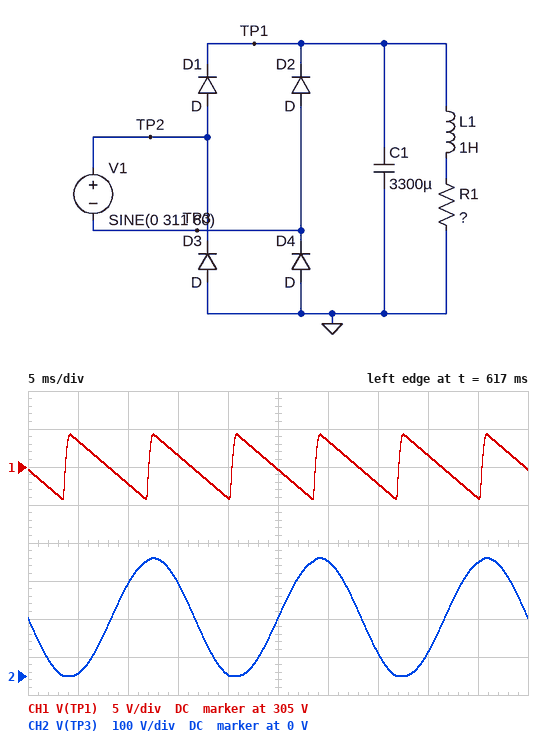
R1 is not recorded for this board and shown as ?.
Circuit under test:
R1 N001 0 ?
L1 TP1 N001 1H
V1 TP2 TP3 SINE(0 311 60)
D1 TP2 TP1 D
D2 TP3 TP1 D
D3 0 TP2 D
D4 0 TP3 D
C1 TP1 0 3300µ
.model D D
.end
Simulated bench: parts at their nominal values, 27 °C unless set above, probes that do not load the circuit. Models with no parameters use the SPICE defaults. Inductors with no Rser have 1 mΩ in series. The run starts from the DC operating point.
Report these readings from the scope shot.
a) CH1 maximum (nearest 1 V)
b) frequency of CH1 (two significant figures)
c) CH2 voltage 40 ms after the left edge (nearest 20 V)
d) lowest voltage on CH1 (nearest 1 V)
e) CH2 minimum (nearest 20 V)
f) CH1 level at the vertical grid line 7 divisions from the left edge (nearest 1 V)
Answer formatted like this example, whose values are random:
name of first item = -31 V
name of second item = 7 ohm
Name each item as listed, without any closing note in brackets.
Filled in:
CH1 maximum = 309 V
frequency of CH1 = 120 Hz
CH2 voltage 40 ms after the left edge = 60 V
lowest voltage on CH1 = 301 V
CH2 minimum = 0 V
CH1 level at the vertical grid line 7 divisions from the left edge = 303 V
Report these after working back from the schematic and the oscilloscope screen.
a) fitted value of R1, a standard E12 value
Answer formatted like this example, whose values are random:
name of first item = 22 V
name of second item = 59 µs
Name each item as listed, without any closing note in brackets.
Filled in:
fitted value of R1, a standard E12 value = 82 Ω
